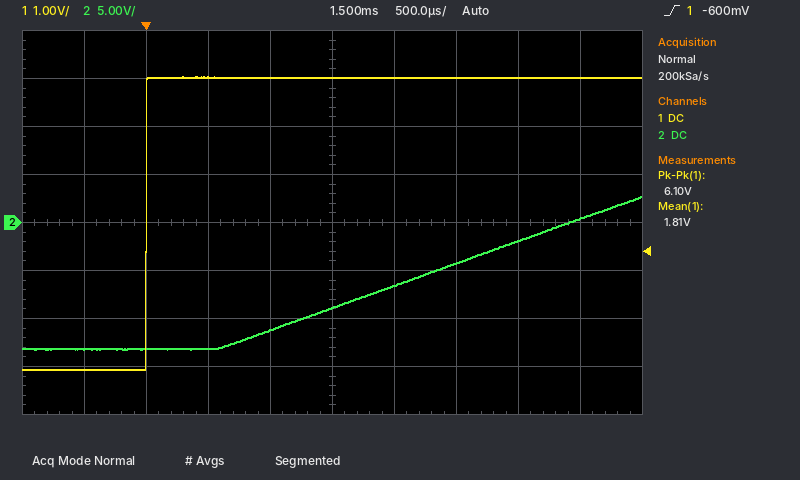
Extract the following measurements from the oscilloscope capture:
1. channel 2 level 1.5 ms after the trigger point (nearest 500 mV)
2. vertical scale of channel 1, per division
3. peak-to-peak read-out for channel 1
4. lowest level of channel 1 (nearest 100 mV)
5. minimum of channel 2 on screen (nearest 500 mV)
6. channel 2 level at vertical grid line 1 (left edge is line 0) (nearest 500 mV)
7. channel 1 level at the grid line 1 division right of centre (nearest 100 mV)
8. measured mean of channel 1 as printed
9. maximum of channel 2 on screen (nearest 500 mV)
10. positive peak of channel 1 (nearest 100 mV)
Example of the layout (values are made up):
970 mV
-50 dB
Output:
-9.0 V
1 V
6.10 V
-3.1 V
-13.0 V
-13.0 V
3.0 V
1.81 V
2.5 V
3.0 V
